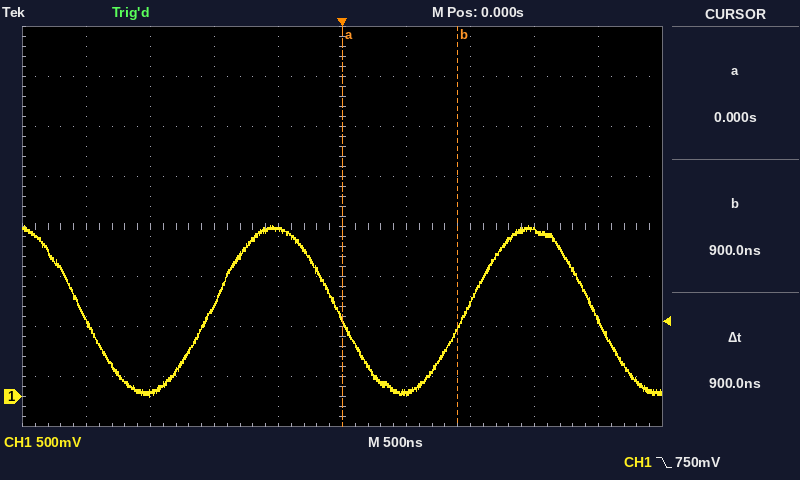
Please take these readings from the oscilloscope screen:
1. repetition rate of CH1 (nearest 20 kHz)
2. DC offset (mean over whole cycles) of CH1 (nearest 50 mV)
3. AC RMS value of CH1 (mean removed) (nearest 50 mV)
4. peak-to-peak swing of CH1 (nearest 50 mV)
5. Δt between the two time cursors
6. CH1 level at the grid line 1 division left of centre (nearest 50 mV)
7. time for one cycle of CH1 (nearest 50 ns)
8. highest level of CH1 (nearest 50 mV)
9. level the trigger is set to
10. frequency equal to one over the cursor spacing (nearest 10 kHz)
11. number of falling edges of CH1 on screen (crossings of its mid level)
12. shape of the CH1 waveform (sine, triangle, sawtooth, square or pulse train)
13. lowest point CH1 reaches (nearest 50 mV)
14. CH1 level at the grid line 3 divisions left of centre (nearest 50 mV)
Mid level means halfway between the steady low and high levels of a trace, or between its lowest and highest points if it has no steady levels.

500 kHz
850 mV
600 mV
1.70 V
900 ns
1.65 V
2.00 µs
1.70 V
750 mV
1.11 MHz
3
sine
0 mV
50 mV
